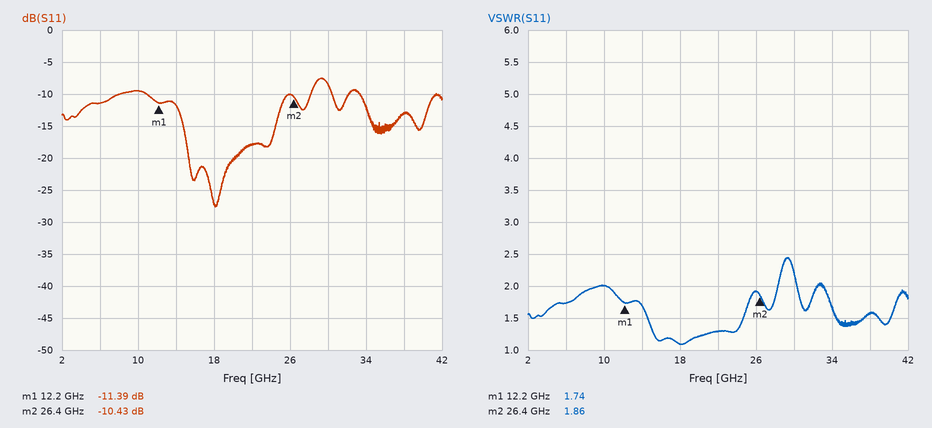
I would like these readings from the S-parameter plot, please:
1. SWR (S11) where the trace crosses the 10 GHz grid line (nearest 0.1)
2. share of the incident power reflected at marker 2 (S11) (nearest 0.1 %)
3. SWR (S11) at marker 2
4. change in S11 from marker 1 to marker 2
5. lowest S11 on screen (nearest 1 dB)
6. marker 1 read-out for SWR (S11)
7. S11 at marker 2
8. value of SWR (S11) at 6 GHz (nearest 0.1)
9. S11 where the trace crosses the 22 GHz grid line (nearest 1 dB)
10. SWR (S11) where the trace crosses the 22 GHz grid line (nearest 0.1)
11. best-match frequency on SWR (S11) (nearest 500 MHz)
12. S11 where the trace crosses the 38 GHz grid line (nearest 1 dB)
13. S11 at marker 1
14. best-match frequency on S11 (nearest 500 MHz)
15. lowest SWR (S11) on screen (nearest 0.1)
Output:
2.0
9.1 %
1.86
0.96 dB
-28 dB
1.74
-10.43 dB
1.7
-18 dB
1.3
18.0 GHz
-13 dB
-11.39 dB
18.0 GHz
1.1
